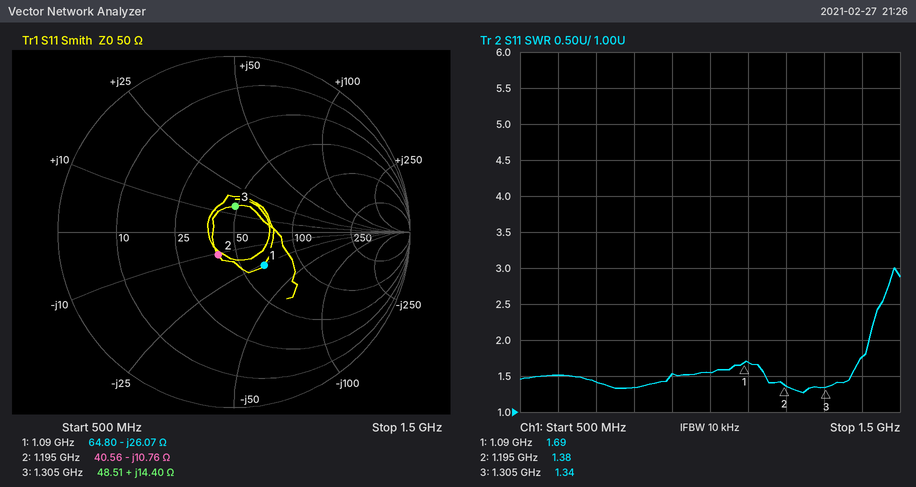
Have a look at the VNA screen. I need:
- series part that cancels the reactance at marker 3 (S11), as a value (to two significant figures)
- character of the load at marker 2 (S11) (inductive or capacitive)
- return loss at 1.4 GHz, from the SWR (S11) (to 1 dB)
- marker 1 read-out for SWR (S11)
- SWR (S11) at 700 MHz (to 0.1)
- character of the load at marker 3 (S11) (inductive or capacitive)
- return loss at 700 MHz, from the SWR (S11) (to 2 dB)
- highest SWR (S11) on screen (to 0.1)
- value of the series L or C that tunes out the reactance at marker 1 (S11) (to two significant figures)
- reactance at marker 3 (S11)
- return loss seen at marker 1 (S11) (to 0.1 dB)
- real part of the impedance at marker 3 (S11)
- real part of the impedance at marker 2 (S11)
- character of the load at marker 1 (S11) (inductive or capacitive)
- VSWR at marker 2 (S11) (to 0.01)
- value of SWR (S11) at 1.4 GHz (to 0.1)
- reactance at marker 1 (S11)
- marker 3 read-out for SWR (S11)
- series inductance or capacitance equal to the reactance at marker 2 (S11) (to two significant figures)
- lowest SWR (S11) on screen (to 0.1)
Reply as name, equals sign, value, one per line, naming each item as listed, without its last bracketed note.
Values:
series part that cancels the reactance at marker 3 (S11), as a value = 8.5 pF
character of the load at marker 2 (S11) = capacitive
return loss at 1.4 GHz, from the SWR (S11) = 11 dB
marker 1 read-out for SWR = 1.69
SWR (S11) at 700 MHz = 1.4
character of the load at marker 3 (S11) = inductive
return loss at 700 MHz, from the SWR (S11) = 16 dB
highest SWR (S11) on screen = 3.0
value of the series L or C that tunes out the reactance at marker 1 (S11) = 3.8 nH
reactance at marker 3 = +14.40 Ω
return loss seen at marker 1 (S11) = 11.9 dB
real part of the impedance at marker 3 = 48.51 Ω
real part of the impedance at marker 2 = 40.56 Ω
character of the load at marker 1 (S11) = capacitive
VSWR at marker 2 (S11) = 1.37
value of SWR (S11) at 1.4 GHz = 1.8
reactance at marker 1 = -26.07 Ω
marker 3 read-out for SWR = 1.34
series inductance or capacitance equal to the reactance at marker 2 (S11) = 12 pF
lowest SWR (S11) on screen = 1.3
